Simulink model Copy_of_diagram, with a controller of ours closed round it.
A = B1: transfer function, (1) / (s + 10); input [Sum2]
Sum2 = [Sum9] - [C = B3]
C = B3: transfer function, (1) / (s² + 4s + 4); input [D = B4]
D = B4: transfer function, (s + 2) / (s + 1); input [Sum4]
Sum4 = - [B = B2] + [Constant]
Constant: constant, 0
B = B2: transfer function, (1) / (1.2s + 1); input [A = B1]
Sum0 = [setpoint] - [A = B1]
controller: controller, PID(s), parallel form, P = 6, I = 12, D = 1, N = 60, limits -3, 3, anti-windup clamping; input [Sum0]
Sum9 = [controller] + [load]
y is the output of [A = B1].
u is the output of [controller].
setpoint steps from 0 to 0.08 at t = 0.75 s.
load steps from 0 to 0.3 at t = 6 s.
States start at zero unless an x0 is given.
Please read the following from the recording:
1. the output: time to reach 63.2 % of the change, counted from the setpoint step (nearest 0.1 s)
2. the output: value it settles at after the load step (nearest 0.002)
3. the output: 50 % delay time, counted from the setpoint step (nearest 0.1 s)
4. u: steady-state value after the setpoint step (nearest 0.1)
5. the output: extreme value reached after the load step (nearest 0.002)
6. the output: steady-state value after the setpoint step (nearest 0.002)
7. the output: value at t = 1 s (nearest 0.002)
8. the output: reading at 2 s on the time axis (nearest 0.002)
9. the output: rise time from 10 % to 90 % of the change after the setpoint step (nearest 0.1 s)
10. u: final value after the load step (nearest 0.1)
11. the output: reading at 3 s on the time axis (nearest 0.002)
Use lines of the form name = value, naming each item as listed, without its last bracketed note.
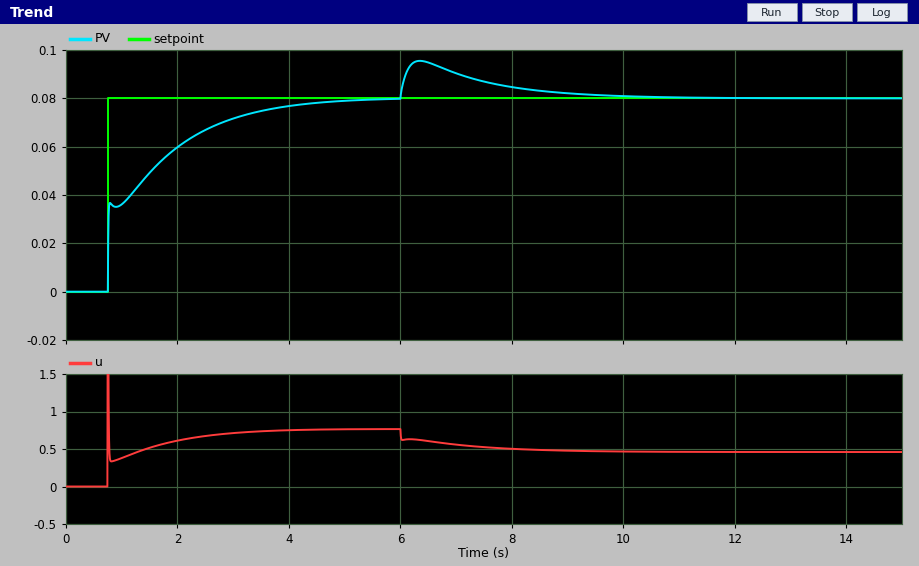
the output: time to reach 63.2 % of the change, counted from the setpoint step = 0.8 s
the output: value it settles at after the load step = 0.080
the output: 50 % delay time, counted from the setpoint step = 0.4 s
u: steady-state value after the setpoint step = 0.8
the output: extreme value reached after the load step = 0.096
the output: steady-state value after the setpoint step = 0.080
the output: value at t = 1 s = 0.036
the output: reading at 2 s on the time axis = 0.060
the output: rise time from 10 % to 90 % of the change after the setpoint step = 2.3 s
u: final value after the load step = 0.5
the output: reading at 3 s on the time axis = 0.072
